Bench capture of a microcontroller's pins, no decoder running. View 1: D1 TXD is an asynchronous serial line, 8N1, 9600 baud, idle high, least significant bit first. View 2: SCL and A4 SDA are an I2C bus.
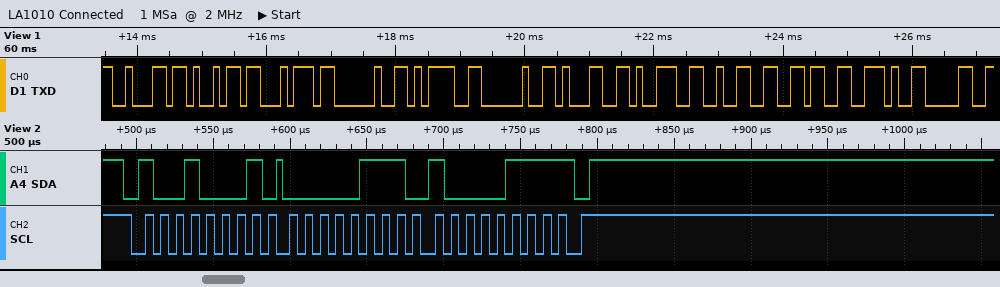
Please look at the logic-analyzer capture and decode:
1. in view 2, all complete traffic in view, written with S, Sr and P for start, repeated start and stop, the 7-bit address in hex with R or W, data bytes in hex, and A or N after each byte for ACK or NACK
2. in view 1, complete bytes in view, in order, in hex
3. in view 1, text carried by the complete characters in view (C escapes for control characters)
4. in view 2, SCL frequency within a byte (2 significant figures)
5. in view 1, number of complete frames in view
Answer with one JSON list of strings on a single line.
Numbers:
["S 48R A 07 A 87 N P", "0x62 0x69 0x74 0x20 0x3D 0x20 0x31 0x39 0x32 0x36 0x2E 0x30", "\"bit = 1926.0\"", "100 kHz", "12"]
